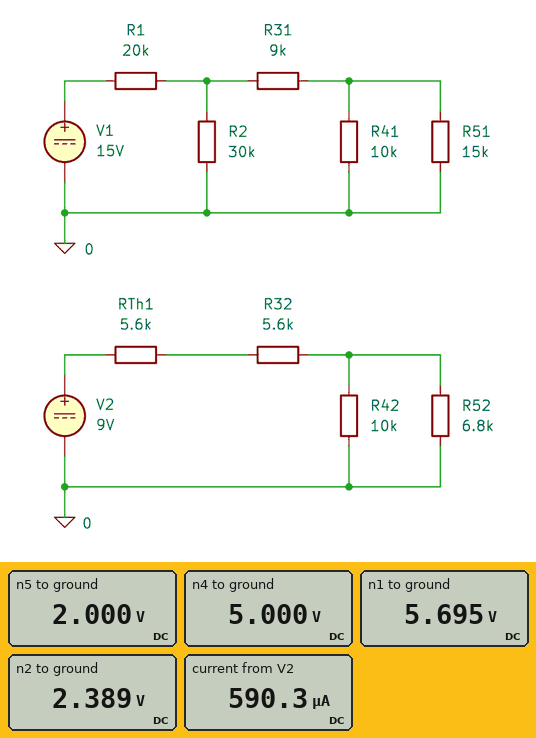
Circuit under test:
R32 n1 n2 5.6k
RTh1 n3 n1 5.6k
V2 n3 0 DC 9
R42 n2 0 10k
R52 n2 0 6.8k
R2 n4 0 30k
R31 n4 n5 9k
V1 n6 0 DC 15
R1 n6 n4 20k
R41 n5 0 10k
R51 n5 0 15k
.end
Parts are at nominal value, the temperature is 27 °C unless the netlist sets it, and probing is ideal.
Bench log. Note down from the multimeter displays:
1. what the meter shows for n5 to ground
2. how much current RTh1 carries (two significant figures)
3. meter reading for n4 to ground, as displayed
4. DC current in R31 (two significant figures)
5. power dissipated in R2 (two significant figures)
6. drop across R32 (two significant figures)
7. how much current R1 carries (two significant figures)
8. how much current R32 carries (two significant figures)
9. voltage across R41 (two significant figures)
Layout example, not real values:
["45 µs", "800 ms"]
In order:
["2.000 V", "590 µA", "5.000 V", "330 µA", "830 µW", "3.3 V", "500 µA", "590 µA", "2.0 V"]
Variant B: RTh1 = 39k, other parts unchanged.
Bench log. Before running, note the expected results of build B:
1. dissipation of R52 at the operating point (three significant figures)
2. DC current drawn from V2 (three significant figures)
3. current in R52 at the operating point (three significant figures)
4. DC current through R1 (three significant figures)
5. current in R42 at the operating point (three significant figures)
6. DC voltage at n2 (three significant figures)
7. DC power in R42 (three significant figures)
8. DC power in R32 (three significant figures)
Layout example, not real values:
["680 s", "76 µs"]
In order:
["82.5 µW", "185 µA", "110 µA", "500 µA", "74.9 µA", "749 mV", "56.1 µW", "192 µW"]
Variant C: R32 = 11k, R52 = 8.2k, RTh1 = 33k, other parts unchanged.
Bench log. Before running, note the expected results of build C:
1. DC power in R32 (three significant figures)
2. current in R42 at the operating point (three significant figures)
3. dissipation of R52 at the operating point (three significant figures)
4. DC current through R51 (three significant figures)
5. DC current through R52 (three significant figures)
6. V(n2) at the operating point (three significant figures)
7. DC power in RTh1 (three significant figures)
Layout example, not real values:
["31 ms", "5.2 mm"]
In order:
["379 µW", "83.6 µA", "85.2 µW", "133 µA", "102 µA", "836 mV", "1.14 mW"]
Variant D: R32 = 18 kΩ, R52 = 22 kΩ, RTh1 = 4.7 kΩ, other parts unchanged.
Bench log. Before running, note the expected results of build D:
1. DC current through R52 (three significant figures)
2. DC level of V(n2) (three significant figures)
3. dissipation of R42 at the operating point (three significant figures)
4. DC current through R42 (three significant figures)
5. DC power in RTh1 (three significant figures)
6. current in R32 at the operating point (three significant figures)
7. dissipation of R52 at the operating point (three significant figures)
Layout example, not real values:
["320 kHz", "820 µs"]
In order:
["95.1 µA", "2.09 V", "438 µW", "209 µA", "435 µW", "304 µA", "199 µW"]
